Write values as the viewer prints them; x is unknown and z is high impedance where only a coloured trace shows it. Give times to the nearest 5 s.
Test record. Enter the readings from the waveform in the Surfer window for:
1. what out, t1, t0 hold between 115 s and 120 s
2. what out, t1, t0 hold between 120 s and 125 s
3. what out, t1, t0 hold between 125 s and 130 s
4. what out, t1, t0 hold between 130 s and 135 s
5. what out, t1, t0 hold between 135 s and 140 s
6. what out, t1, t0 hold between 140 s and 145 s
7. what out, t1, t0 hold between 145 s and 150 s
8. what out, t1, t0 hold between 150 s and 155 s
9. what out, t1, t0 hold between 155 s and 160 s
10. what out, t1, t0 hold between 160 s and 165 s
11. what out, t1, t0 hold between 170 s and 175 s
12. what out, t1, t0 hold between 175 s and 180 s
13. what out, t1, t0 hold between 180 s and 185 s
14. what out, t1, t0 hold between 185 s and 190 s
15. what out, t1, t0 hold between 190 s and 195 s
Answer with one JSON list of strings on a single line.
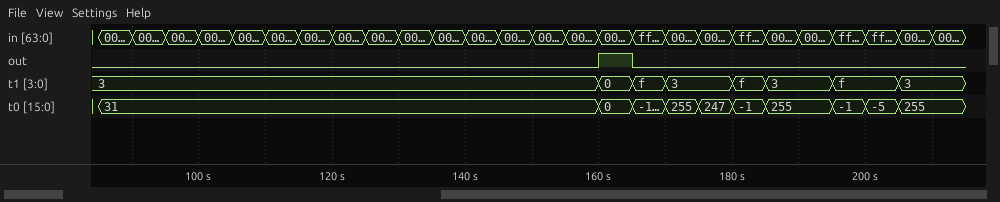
["out=0, t1=3, t0=31", "out=0, t1=3, t0=31", "out=0, t1=3, t0=31", "out=0, t1=3, t0=31", "out=0, t1=3, t0=31", "out=0, t1=3, t0=31", "out=0, t1=3, t0=31", "out=0, t1=3, t0=31", "out=0, t1=3, t0=31", "out=1, t1=0, t0=0", "out=0, t1=3, t0=255", "out=0, t1=3, t0=247", "out=0, t1=f, t0=-1", "out=0, t1=3, t0=255", "out=0, t1=3, t0=255"]
